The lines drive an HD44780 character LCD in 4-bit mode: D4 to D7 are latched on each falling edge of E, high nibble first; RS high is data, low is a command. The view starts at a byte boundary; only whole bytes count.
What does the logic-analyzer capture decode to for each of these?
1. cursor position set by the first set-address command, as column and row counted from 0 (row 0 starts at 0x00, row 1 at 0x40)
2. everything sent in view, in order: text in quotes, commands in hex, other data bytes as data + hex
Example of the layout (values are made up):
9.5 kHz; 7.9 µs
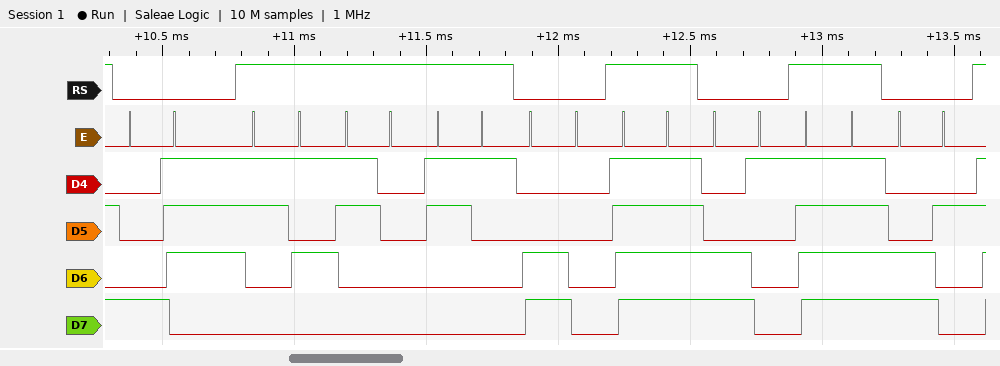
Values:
column 7, row 0; 0x87 "501" 0xC0 data FF 0xC1 data FF 0xC2
